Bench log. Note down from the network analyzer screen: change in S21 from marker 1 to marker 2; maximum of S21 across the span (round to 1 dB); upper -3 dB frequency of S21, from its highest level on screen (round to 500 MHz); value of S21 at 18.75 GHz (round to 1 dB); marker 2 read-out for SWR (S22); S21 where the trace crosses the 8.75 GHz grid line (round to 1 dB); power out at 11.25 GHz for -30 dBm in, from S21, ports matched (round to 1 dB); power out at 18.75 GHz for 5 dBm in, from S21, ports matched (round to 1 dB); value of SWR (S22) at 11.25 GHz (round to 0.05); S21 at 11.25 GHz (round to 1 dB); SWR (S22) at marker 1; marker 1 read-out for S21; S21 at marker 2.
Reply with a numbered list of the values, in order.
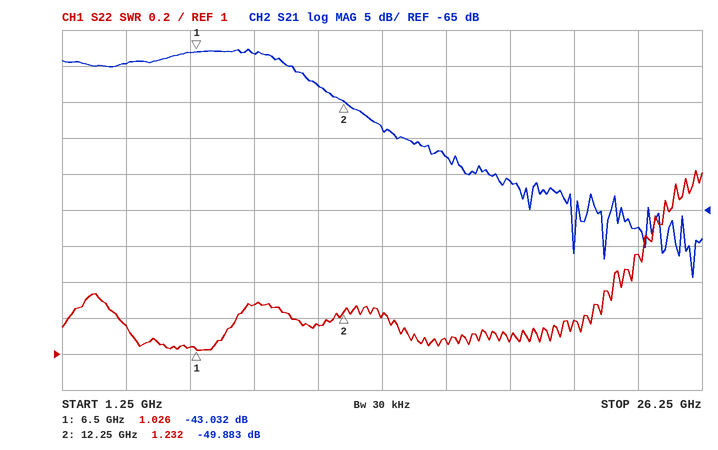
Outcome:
1. -6.851 dB
2. -43 dB
3. 10.5 GHz
4. -61 dB
5. 1.232
6. -43 dB
7. -78 dBm
8. -56 dBm
9. 1.15
10. -48 dB
11. 1.026
12. -43.032 dB
13. -49.883 dB
